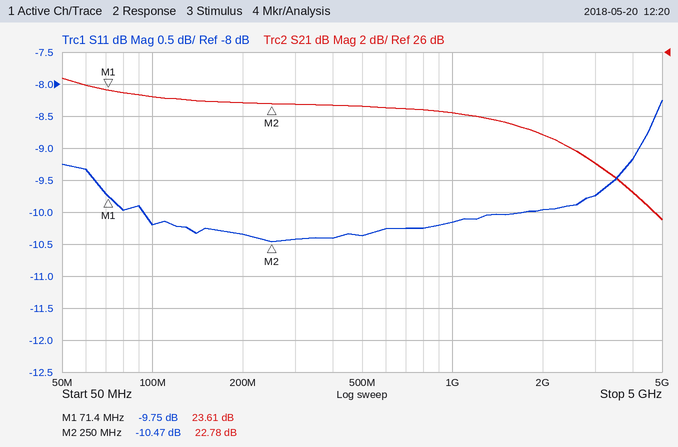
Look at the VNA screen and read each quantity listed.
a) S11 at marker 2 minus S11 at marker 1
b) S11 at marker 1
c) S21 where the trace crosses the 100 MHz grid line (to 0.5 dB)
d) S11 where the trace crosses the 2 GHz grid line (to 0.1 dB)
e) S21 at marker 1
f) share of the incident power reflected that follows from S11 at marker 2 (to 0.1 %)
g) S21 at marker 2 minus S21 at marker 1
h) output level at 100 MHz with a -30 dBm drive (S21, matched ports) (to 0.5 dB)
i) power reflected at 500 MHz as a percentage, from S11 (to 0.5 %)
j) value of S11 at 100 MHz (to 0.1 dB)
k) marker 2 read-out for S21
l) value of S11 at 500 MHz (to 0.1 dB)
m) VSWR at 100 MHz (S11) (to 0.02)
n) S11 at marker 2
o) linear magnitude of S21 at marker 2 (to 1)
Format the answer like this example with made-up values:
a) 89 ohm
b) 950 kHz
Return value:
a) -0.72 dB
b) -9.75 dB
c) 23.0 dB
d) -10.0 dB
e) 23.61 dB
f) 9.0 %
g) -0.83 dB
h) -7.0 dBm
i) 9.0 %
j) -10.2 dB
k) 22.78 dB
l) -10.4 dB
m) 1.90
n) -10.47 dB
o) 14
